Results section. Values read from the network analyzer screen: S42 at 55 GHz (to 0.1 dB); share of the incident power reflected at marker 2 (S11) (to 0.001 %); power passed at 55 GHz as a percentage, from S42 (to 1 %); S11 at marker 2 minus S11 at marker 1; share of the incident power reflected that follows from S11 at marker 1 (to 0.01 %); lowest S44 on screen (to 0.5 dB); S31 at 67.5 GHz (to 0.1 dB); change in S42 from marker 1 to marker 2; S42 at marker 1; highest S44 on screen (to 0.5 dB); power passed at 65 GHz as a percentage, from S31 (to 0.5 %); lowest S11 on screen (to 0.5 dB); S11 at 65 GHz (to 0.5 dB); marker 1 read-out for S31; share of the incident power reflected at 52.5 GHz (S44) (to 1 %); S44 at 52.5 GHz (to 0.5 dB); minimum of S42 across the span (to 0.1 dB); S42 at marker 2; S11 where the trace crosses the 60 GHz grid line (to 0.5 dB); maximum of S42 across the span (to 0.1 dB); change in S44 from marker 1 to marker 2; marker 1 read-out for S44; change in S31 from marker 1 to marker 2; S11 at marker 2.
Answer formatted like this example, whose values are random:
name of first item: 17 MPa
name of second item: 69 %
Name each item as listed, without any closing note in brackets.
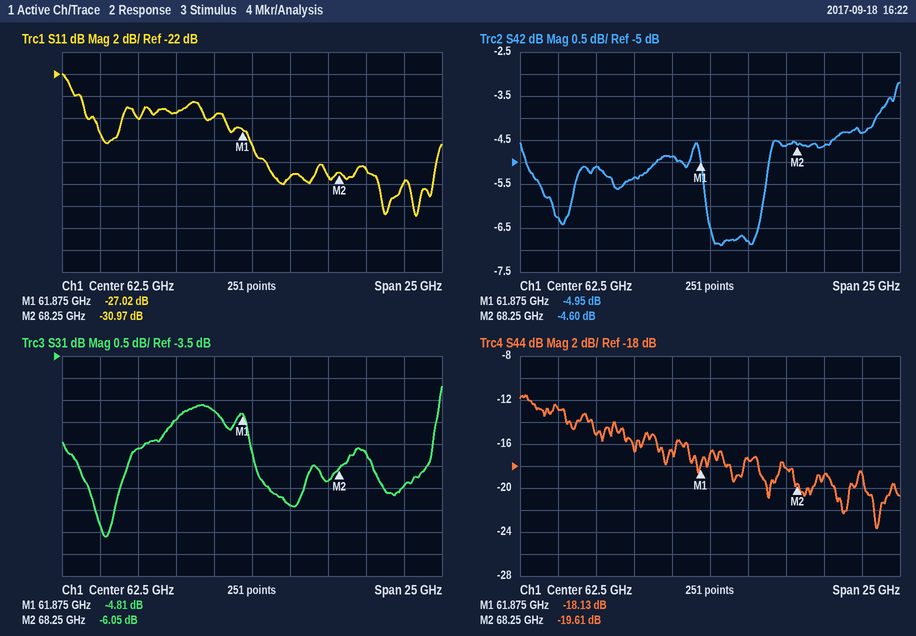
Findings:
S42 at 55 GHz: -5.1 dB
share of the incident power reflected at marker 2 (S11): 0.080 %
power passed at 55 GHz as a percentage, from S42: 31 %
S11 at marker 2 minus S11 at marker 1: -3.95 dB
share of the incident power reflected that follows from S11 at marker 1: 0.20 %
lowest S44 on screen: -23.5 dB
S31 at 67.5 GHz: -6.3 dB
change in S42 from marker 1 to marker 2: 0.35 dB
S42 at marker 1: -4.95 dB
highest S44 on screen: -11.5 dB
power passed at 65 GHz as a percentage, from S31: 20.5 %
lowest S11 on screen: -35.0 dB
S11 at 65 GHz: -31.5 dB
marker 1 read-out for S31: -4.81 dB
share of the incident power reflected at 52.5 GHz (S44): 5 %
S44 at 52.5 GHz: -13.0 dB
minimum of S42 across the span: -6.9 dB
S42 at marker 2: -4.60 dB
S11 where the trace crosses the 60 GHz grid line: -26.0 dB
maximum of S42 across the span: -3.2 dB
change in S44 from marker 1 to marker 2: -1.48 dB
marker 1 read-out for S44: -18.13 dB
change in S31 from marker 1 to marker 2: -1.24 dB
S11 at marker 2: -30.97 dB
